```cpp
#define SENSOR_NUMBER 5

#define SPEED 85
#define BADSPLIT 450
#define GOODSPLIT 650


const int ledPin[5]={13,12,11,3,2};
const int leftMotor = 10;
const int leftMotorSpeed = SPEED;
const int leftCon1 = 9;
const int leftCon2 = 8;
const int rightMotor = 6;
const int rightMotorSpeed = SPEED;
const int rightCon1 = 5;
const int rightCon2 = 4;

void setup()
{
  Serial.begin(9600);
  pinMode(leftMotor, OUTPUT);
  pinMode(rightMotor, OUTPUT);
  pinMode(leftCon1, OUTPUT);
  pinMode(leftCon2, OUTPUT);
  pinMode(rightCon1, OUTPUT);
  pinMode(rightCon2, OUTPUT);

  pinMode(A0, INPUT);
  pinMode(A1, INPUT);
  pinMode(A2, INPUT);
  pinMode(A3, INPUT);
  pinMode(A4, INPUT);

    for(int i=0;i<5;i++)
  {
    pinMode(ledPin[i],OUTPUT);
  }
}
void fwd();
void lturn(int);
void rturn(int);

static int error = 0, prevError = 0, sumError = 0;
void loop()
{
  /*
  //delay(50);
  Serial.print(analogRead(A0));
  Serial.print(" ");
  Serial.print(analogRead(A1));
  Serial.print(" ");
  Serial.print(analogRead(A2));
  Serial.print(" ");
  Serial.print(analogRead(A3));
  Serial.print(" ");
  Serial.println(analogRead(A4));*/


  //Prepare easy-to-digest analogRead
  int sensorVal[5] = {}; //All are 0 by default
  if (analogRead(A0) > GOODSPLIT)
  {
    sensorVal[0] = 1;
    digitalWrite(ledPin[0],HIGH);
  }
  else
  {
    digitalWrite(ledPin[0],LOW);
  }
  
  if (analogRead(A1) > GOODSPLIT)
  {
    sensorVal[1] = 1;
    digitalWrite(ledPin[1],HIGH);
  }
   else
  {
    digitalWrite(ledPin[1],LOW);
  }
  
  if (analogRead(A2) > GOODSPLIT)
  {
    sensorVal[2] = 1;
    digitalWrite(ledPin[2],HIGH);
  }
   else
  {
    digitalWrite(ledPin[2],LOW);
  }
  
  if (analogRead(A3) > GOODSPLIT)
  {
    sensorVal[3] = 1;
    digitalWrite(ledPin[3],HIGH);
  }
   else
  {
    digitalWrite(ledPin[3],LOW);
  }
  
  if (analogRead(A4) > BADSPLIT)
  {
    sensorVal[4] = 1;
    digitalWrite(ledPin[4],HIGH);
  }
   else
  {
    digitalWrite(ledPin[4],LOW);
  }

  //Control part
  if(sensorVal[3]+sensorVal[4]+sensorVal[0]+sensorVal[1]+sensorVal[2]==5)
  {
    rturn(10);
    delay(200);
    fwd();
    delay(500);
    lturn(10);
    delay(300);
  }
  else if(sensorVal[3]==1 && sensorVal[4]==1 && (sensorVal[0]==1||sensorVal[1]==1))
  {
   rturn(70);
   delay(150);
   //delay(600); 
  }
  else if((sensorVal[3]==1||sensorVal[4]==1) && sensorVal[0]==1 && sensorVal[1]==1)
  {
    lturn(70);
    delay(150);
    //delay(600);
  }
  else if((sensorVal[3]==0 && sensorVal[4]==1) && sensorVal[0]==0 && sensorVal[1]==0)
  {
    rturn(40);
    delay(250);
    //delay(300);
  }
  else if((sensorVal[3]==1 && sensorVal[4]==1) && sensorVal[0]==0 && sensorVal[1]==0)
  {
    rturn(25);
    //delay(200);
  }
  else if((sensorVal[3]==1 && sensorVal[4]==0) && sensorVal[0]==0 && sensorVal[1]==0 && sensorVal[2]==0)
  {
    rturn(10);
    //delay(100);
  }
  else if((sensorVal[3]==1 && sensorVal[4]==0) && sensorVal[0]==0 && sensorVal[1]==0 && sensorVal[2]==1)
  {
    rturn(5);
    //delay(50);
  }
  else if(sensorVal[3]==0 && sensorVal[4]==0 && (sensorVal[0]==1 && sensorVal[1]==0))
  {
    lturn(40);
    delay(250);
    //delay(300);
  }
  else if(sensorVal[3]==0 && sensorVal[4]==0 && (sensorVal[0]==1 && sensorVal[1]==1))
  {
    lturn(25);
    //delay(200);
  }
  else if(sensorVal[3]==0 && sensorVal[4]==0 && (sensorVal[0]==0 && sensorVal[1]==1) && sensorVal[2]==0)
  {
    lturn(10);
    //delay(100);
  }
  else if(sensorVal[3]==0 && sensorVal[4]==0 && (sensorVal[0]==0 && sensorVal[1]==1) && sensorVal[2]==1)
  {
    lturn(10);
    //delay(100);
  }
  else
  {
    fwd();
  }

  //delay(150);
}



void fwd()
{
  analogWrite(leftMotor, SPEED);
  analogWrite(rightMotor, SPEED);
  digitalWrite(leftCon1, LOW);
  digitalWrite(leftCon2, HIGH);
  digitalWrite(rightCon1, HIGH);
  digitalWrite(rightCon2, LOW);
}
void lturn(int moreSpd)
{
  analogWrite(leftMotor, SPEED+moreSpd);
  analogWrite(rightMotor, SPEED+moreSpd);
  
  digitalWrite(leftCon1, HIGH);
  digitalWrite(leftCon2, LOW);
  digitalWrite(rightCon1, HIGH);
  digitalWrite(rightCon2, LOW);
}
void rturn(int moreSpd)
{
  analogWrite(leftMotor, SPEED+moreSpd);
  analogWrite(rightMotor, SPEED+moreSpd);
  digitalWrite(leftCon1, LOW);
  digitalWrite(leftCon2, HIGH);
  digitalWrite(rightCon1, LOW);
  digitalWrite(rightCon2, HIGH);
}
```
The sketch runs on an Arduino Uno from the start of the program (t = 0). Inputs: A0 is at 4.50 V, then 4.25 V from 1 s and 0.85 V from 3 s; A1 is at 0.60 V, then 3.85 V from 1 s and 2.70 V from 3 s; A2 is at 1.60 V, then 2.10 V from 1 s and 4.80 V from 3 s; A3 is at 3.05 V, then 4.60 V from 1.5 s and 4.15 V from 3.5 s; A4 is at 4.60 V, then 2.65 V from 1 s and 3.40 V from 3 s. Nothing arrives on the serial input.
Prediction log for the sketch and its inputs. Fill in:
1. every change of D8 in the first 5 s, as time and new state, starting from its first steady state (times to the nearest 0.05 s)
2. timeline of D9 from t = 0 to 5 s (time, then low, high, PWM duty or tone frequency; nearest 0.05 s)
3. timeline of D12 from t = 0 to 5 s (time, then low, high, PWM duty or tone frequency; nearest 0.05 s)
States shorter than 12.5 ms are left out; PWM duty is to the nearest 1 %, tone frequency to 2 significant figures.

0 s high; 1 s low; 1.6 s high
0 s low; 1 s high; 1.6 s low
0 s low; 1 s high; 3.1 s low
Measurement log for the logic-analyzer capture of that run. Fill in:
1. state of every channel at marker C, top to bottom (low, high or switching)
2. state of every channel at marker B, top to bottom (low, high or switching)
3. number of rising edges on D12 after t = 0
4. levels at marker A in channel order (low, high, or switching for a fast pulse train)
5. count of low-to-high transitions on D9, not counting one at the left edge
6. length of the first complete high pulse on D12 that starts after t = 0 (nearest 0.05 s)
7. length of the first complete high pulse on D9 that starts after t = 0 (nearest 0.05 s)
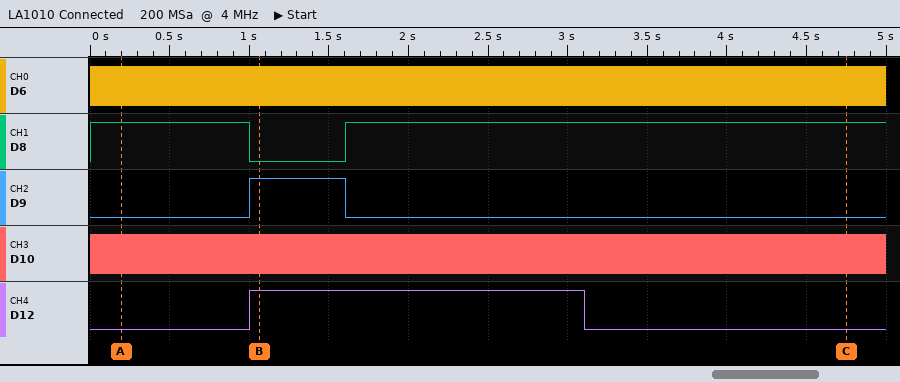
D6 switching, D8 high, D9 low, D10 switching, D12 low
D6 switching, D8 low, D9 high, D10 switching, D12 high
1
D6 switching, D8 high, D9 low, D10 switching, D12 low
1
2.10 s
0.60 s
